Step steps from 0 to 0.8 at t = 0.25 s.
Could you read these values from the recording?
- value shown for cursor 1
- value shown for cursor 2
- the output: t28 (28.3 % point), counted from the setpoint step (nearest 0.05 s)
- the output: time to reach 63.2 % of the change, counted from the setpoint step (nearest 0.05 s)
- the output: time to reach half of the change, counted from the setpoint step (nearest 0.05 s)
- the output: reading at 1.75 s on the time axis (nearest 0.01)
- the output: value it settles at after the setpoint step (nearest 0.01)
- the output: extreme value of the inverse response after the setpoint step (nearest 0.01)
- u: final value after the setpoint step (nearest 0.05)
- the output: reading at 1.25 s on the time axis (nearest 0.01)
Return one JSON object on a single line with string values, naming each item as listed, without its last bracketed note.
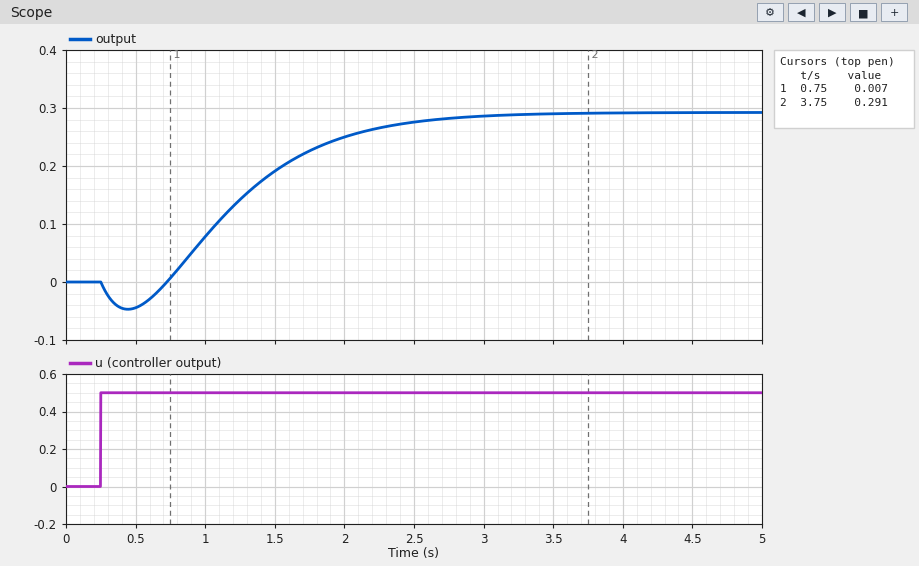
{"value shown for cursor 1": "0.007", "value shown for cursor 2": "0.291", "the output: t28 (28.3 % point), counted from the setpoint step": "0.75 s", "the output: time to reach 63.2 % of the change, counted from the setpoint step": "1.20 s", "the output: time to reach half of the change, counted from the setpoint step": "1.00 s", "the output: reading at 1.75 s on the time axis": "0.23", "the output: value it settles at after the setpoint step": "0.29", "the output: extreme value of the inverse response after the setpoint step": "-0.05", "u: final value after the setpoint step": "0.50", "the output: reading at 1.25 s on the time axis": "0.14"}
